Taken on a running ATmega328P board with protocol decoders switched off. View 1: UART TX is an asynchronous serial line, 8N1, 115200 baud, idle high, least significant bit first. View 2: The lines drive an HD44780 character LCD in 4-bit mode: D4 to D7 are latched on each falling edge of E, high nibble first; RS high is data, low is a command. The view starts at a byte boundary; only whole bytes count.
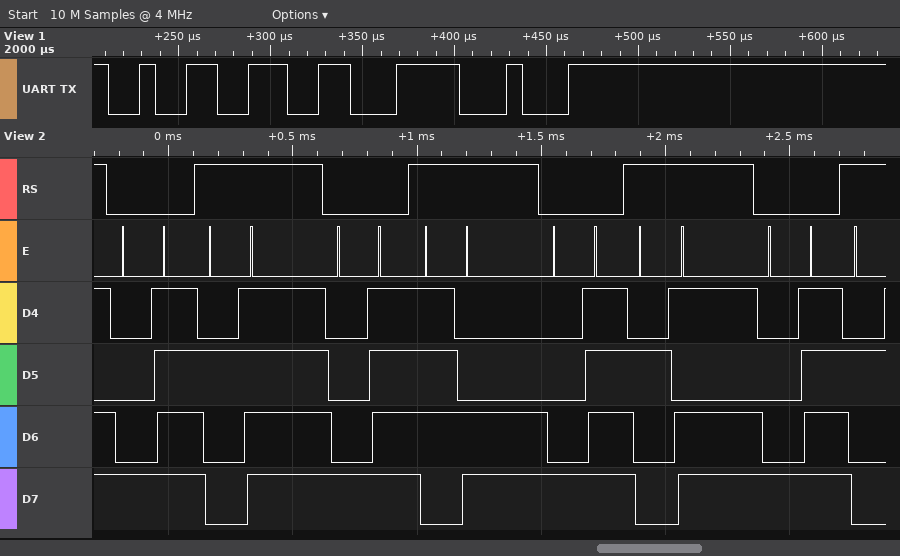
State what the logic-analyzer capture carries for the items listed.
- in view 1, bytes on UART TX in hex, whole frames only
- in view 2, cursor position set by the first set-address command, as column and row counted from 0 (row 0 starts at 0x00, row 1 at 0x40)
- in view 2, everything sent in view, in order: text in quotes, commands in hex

32 C6 C4
column 15, row 0
0x8F "/" 0x8F "|" 0x8F "-" 0x8F
